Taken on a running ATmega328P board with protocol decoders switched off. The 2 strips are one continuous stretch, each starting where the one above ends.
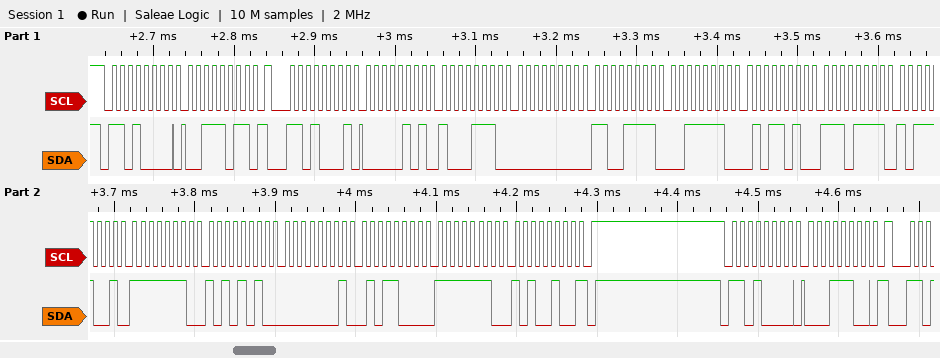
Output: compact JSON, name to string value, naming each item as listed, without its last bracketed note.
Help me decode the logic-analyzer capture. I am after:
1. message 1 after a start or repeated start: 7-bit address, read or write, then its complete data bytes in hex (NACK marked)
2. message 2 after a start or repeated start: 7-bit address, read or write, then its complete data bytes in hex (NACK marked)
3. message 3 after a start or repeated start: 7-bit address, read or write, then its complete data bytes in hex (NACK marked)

{"message 1 after a start or repeated start: 7-bit address, read or write, then its complete data bytes in hex": "0x68 write: 3B", "message 2 after a start or repeated start: 7-bit address, read or write, then its complete data bytes in hex": "0x68 read: 05 8E 00 CF 3E 5A EF B9 FE AA 01 58 FE A4 NACK", "message 3 after a start or repeated start: 7-bit address, read or write, then its complete data bytes in hex": "0x68 write: 1C"}
